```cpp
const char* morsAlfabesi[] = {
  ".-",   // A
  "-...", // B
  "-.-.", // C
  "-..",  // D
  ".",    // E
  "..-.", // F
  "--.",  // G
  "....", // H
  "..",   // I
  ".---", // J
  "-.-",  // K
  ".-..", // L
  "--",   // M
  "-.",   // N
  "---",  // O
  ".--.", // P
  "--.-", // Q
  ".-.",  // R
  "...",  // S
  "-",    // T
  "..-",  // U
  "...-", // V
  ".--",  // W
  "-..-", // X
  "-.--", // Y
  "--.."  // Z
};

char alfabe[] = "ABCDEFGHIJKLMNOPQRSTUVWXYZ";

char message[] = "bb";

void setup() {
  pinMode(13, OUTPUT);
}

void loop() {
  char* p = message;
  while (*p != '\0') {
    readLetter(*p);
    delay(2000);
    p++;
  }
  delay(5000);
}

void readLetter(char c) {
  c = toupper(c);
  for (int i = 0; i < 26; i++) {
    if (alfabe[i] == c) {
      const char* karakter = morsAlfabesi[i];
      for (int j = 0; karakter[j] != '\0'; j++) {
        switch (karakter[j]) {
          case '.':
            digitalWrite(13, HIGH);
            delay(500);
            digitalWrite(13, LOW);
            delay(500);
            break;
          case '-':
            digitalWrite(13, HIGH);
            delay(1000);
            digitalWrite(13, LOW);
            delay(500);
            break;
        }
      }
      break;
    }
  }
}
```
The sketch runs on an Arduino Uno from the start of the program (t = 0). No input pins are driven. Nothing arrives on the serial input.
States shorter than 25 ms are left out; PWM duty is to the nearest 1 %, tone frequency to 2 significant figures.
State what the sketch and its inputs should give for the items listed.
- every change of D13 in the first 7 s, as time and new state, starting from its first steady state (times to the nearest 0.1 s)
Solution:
0 s high; 1 s low; 1.5 s high; 2 s low; 2.5 s high; 3 s low; 3.5 s high; 4 s low; 6.5 s high
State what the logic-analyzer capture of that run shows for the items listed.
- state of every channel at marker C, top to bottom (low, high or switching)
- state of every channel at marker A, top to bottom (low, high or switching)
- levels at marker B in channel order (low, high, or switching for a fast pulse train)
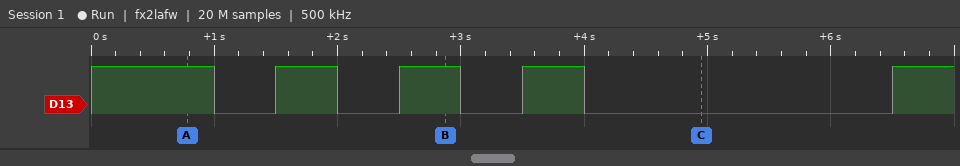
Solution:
D13 low
D13 high
D13 high
